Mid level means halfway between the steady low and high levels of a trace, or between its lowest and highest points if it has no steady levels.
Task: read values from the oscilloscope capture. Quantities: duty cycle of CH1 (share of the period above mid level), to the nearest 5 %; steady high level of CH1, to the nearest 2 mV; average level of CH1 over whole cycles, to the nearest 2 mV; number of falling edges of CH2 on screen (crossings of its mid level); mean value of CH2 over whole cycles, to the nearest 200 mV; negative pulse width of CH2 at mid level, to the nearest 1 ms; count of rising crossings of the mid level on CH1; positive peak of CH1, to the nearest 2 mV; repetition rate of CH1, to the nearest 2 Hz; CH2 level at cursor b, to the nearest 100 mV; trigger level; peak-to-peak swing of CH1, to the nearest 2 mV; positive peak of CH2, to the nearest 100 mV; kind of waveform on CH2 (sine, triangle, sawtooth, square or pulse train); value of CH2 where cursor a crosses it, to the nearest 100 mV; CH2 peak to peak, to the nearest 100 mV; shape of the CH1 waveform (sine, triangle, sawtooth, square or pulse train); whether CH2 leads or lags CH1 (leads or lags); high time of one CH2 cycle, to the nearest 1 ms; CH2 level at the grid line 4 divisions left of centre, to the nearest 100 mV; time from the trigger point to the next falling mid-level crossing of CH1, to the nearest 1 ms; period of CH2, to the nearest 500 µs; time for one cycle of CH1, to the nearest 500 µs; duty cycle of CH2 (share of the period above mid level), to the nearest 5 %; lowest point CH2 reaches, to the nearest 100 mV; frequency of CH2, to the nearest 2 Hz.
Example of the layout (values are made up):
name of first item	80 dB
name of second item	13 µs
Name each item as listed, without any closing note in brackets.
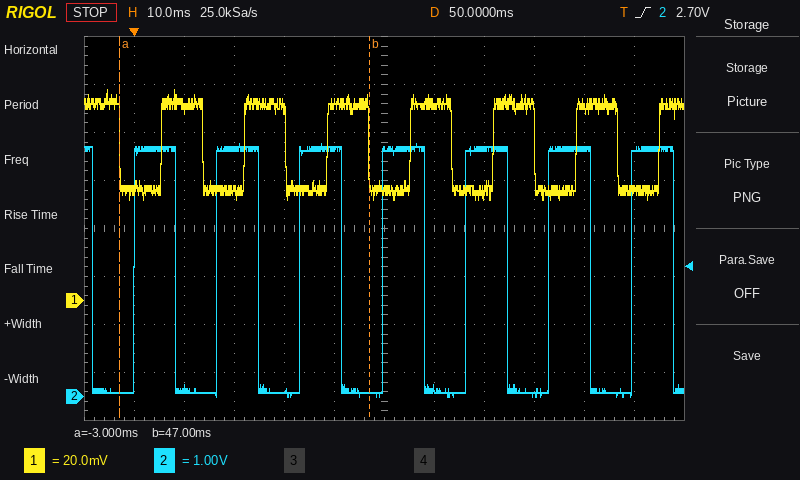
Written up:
duty cycle of CH1 (share of the period above mid level), to the nearest 5 %	50 %
steady high level of CH1, to the nearest 2 mV	82 mV
average level of CH1 over whole cycles, to the nearest 2 mV	64 mV
number of falling edges of CH2 on screen	8
mean value of CH2 over whole cycles, to the nearest 200 mV	2.6 V
negative pulse width of CH2 at mid level, to the nearest 1 ms	8 ms
count of rising crossings of the mid level on CH1	7
positive peak of CH1, to the nearest 2 mV	88 mV
repetition rate of CH1, to the nearest 2 Hz	60 Hz
CH2 level at cursor b, to the nearest 100 mV	100 mV
trigger level	2.70 V
peak-to-peak swing of CH1, to the nearest 2 mV	46 mV
positive peak of CH2, to the nearest 100 mV	5.3 V
kind of waveform on CH2	square
value of CH2 where cursor a crosses it, to the nearest 100 mV	100 mV
CH2 peak to peak, to the nearest 100 mV	5.3 V
shape of the CH1 waveform	square
whether CH2 leads or lags CH1	leads
high time of one CH2 cycle, to the nearest 1 ms	8 ms
CH2 level at the grid line 4 divisions left of centre, to the nearest 100 mV	200 mV
time from the trigger point to the next falling mid-level crossing of CH1, to the nearest 1 ms	14 ms
period of CH2, to the nearest 500 µs	16.5 ms
time for one cycle of CH1, to the nearest 500 µs	16.5 ms
duty cycle of CH2 (share of the period above mid level), to the nearest 5 %	50 %
lowest point CH2 reaches, to the nearest 100 mV	0.0 V
frequency of CH2, to the nearest 2 Hz	60 Hz
